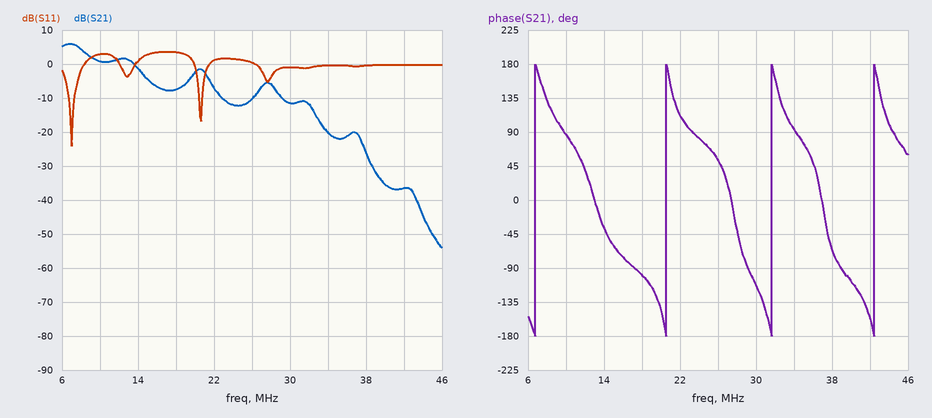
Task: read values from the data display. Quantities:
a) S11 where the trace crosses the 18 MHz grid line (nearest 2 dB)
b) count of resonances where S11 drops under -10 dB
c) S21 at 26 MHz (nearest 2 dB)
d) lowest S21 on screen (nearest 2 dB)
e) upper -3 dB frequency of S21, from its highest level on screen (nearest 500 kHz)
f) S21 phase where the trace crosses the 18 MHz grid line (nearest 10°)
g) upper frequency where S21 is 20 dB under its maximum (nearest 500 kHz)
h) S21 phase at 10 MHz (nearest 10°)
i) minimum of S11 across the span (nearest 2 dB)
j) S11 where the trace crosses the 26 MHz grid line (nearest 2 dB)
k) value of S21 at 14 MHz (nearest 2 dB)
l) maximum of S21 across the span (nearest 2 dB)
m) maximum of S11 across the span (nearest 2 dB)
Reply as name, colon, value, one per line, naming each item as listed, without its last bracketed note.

S11 where the trace crosses the 18 MHz grid line: 4 dB
count of resonances where S11 drops under -10 dB: 2
S21 at 26 MHz: -10 dB
lowest S21 on screen: -54 dB
upper -3 dB frequency of S21, from its highest level on screen: 8.5 MHz
S21 phase where the trace crosses the 18 MHz grid line: -100°
upper frequency where S21 is 20 dB under its maximum: 32.5 MHz
S21 phase at 10 MHz: 90°
minimum of S11 across the span: -24 dB
S11 where the trace crosses the 26 MHz grid line: 0 dB
value of S21 at 14 MHz: -2 dB
maximum of S21 across the span: 6 dB
maximum of S11 across the span: 4 dB
